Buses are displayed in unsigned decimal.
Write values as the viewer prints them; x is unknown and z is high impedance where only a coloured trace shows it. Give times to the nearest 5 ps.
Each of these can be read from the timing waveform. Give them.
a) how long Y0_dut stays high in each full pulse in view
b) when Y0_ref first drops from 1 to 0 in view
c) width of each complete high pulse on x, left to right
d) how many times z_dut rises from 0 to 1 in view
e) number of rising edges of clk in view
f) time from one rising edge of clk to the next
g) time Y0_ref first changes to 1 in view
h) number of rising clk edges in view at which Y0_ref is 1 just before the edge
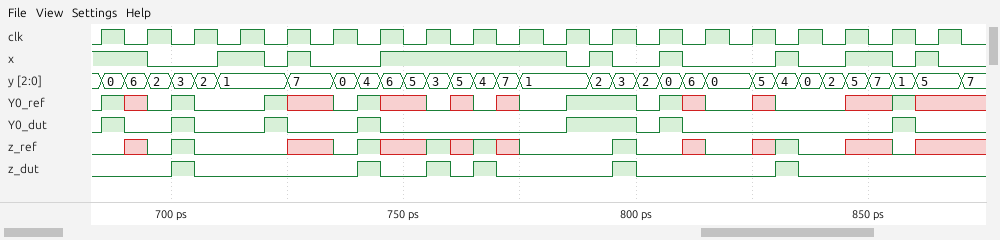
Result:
5 ps, 5 ps, 5 ps, 5 ps, 15 ps, 5 ps, 5 ps
705 ps
10 ps, 5 ps, 40 ps, 5 ps, 5 ps, 5 ps, 10 ps, 5 ps
6
19
10 ps
685 ps
4
